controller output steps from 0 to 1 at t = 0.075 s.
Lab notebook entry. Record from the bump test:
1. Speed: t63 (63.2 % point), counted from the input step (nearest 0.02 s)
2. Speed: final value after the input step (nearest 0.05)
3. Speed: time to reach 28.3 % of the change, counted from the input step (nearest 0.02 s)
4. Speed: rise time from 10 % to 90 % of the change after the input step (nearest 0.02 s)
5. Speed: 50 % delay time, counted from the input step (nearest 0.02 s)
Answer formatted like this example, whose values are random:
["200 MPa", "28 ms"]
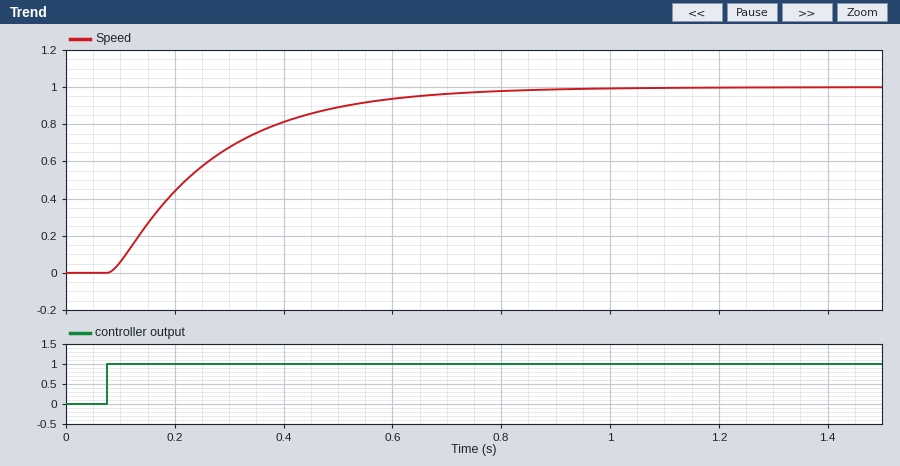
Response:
["0.20 s", "1.00", "0.08 s", "0.40 s", "0.14 s"]
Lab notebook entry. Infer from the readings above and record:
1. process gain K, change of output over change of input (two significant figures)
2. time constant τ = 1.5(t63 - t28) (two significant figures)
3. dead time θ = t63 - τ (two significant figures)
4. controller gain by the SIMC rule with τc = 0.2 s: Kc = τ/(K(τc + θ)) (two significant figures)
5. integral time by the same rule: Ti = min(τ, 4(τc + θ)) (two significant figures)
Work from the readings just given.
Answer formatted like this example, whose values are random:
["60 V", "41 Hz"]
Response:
["1.0", "0.18 s", "0.020 s", "0.82", "0.18 s"]
